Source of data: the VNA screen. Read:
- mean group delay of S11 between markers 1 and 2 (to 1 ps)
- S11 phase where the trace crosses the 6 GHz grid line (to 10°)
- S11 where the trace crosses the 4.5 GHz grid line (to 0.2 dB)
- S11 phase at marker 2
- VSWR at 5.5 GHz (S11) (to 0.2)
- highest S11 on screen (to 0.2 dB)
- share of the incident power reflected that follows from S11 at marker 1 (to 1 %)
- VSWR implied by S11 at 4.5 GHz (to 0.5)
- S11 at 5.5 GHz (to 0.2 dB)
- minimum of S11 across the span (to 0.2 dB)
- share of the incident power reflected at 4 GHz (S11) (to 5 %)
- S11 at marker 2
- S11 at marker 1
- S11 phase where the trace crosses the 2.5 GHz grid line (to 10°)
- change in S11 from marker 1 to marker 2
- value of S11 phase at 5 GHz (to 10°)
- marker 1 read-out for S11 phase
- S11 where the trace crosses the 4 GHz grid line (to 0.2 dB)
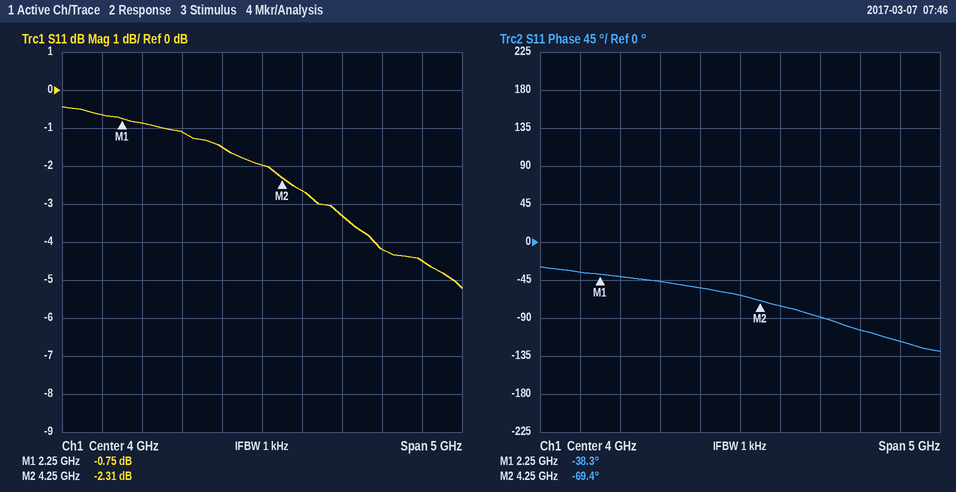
43 ps
-120°
-2.6 dB
-69.4°
4.2
-0.4 dB
84 %
6.5
-4.2 dB
-5.2 dB
65 %
-2.31 dB
-0.75 dB
-40°
-1.56 dB
-90°
-38.3°
-2.0 dB
